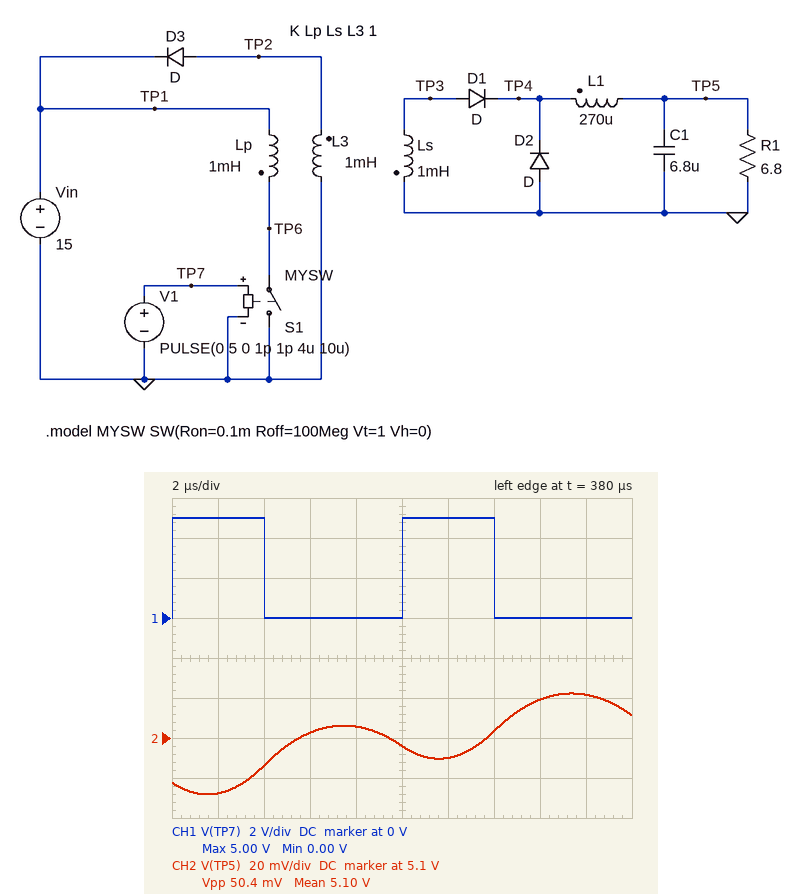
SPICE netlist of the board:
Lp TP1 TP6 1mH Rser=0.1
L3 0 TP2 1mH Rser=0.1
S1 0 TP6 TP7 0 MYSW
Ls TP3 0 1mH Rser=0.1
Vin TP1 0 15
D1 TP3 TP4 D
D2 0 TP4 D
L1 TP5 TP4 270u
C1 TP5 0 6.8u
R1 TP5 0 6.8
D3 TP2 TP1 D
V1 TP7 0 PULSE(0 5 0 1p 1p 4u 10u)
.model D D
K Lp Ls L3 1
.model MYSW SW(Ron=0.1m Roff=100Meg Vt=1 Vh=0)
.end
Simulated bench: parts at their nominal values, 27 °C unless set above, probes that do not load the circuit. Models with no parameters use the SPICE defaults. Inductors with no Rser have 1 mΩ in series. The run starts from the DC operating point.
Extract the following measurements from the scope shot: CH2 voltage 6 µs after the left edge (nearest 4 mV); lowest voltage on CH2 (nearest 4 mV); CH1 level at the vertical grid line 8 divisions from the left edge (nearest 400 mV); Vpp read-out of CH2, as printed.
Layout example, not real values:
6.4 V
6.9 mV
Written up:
5.104 V
5.072 V
0 V
50.4 mV
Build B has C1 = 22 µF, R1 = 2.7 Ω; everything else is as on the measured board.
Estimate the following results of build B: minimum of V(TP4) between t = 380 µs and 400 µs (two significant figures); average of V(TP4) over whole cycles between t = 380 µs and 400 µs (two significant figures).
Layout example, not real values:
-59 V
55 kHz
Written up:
-850 mV
5.0 V
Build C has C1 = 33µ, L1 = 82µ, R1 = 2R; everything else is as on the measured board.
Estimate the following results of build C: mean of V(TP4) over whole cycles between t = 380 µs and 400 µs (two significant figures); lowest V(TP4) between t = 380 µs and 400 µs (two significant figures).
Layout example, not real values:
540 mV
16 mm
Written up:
4.9 V
-860 mV
